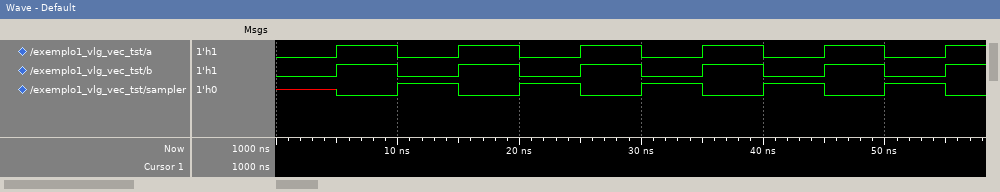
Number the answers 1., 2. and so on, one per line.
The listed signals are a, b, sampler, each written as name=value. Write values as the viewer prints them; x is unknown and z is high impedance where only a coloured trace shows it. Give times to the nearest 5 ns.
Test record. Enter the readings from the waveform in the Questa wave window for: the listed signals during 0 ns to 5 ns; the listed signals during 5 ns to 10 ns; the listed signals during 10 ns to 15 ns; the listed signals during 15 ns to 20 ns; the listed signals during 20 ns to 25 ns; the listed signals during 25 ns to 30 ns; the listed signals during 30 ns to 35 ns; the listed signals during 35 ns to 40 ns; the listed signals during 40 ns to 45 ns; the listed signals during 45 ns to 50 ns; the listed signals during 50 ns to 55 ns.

1. a=0, b=0, sampler=x
2. a=1, b=1, sampler=0
3. a=0, b=0, sampler=1
4. a=1, b=1, sampler=0
5. a=0, b=0, sampler=1
6. a=1, b=1, sampler=0
7. a=0, b=0, sampler=1
8. a=1, b=1, sampler=0
9. a=0, b=0, sampler=1
10. a=1, b=1, sampler=0
11. a=0, b=0, sampler=1
